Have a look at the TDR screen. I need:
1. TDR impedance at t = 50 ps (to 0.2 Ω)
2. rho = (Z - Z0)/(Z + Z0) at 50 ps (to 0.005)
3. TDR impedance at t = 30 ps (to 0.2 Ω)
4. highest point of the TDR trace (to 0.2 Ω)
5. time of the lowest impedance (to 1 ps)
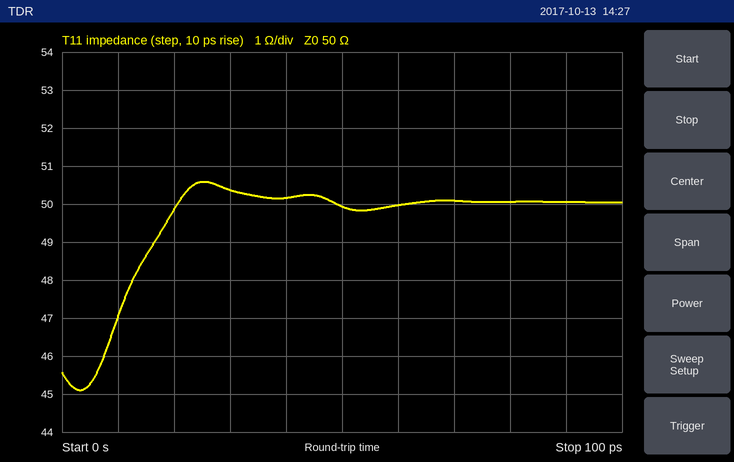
50.0 Ω
0.000
50.4 Ω
50.6 Ω
3 ps
